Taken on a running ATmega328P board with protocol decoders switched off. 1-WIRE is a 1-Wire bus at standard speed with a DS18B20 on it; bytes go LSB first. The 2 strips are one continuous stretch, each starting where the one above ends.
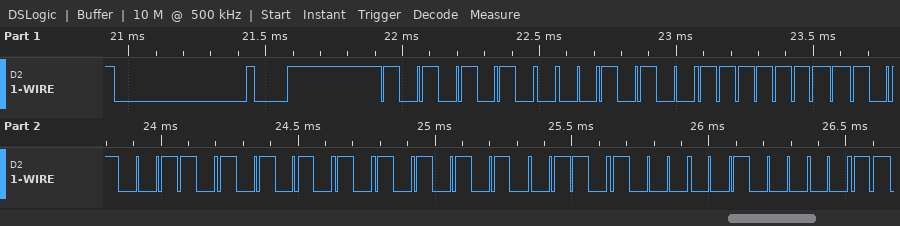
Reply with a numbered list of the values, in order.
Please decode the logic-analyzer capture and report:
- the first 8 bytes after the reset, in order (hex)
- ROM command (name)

1. 55 28 FF 65 55 55 16 04
2. Match ROM
